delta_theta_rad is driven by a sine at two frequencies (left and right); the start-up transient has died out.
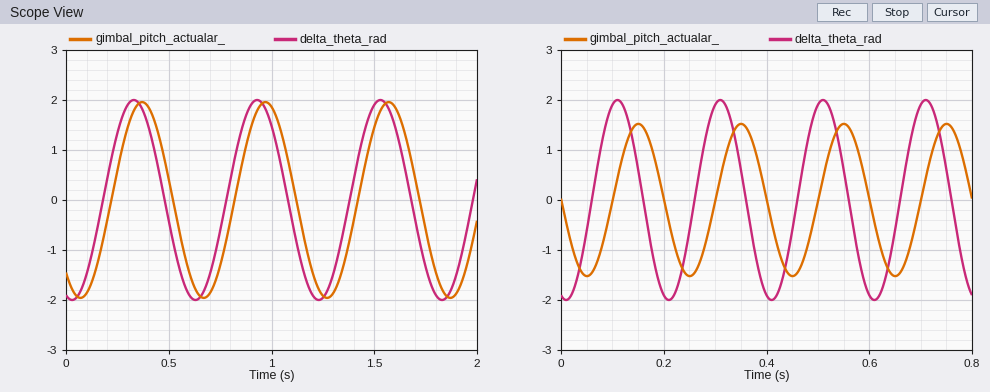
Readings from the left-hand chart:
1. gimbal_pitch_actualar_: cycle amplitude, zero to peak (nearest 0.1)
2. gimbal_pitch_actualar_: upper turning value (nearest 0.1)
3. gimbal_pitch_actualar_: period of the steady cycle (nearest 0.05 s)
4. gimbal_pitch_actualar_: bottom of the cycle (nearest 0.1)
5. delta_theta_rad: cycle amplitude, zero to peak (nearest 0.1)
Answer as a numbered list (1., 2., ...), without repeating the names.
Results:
1. 2.0
2. 2.0
3. 0.60 s
4. -2.0
5. 2.0
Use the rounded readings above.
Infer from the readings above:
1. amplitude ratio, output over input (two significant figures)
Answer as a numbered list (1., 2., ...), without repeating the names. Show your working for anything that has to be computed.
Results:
1. 2 / 2 = 1.0
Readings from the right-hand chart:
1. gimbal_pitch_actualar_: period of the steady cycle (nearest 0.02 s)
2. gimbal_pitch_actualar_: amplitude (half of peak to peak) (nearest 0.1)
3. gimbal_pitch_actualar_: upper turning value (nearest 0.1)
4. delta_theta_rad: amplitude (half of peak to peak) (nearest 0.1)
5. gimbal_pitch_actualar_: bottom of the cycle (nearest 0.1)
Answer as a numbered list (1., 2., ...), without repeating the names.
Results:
1. 0.20 s
2. 1.5
3. 1.5
4. 2.0
5. -1.5
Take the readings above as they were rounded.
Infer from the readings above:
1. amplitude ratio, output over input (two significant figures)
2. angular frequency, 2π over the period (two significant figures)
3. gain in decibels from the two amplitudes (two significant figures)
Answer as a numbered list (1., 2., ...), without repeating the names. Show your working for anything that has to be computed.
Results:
1. 1.5 / 2 = 0.75
2. 2π / 0.2 = 31 rad/s
3. 20 log10(1.5 / 2) = -2.5 dB
